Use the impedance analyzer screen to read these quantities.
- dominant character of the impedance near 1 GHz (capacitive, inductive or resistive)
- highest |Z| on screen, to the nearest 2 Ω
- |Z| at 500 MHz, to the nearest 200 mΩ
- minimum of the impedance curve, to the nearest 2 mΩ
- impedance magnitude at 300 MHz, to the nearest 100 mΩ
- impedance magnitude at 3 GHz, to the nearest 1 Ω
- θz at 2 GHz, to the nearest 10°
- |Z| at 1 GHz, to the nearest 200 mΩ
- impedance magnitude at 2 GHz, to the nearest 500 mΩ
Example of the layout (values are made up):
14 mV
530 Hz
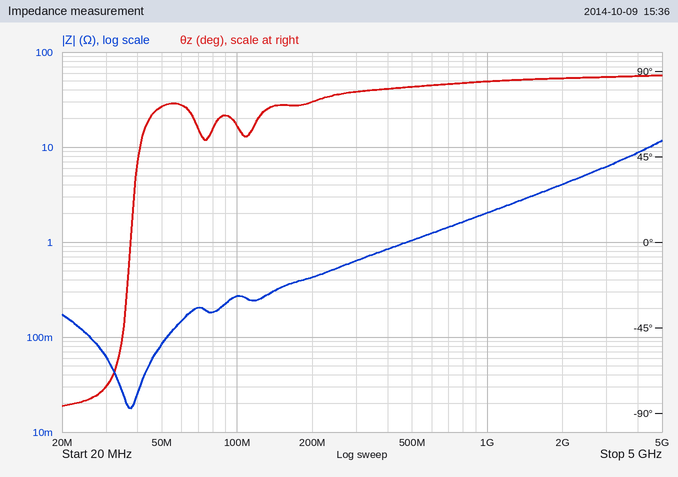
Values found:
inductive
12 Ω
1.0 Ω
18 mΩ
600 mΩ
6 Ω
90°
2.0 Ω
4.0 Ω
